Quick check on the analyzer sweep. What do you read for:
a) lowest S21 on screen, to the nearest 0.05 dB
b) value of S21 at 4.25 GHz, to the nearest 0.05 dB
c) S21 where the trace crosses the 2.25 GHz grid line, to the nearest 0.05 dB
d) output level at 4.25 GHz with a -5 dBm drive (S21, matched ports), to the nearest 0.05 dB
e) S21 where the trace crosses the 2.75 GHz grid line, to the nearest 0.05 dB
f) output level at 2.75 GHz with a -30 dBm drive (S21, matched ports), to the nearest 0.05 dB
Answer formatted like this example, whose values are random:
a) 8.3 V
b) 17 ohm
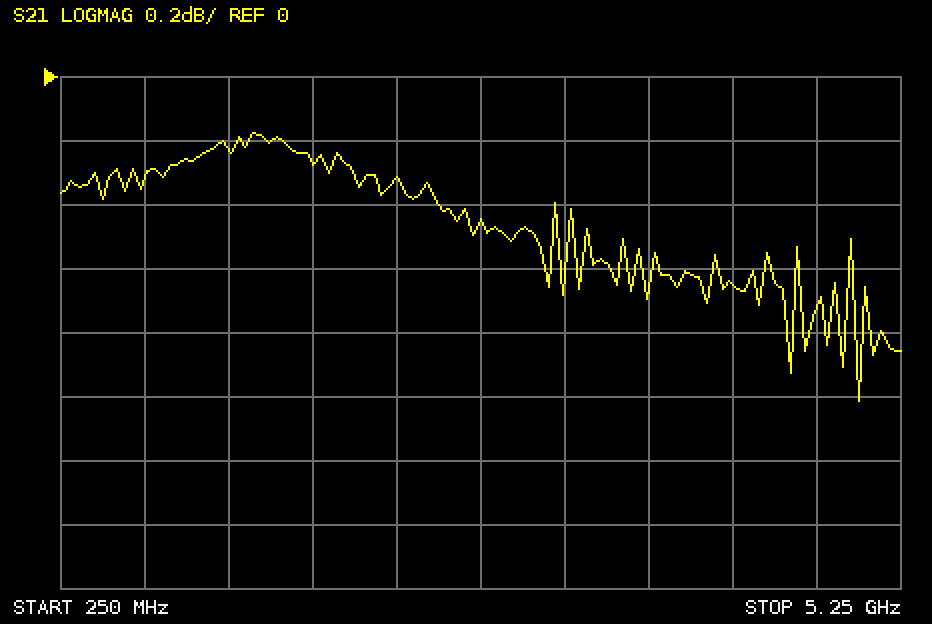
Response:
a) -1.00 dB
b) -0.65 dB
c) -0.30 dB
d) -5.65 dBm
e) -0.45 dB
f) -30.45 dBm
